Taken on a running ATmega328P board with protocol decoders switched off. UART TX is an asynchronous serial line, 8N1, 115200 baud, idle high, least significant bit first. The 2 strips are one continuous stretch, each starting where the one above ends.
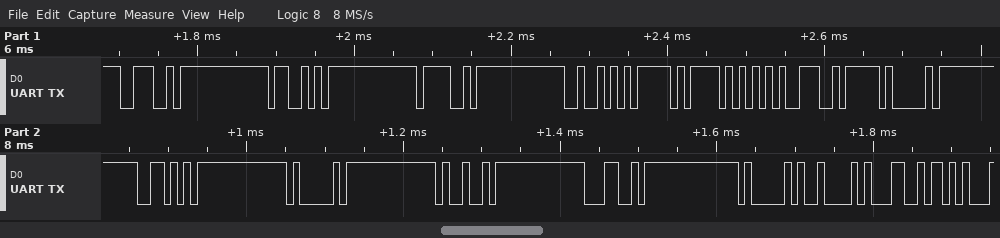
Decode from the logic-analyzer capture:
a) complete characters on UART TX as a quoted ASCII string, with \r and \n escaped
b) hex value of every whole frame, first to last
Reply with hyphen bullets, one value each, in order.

- "NSOR_UNAVAILABL"
- 0x4E 0x53 0x4F 0x52 0x5F 0x55 0x4E 0x41 0x56 0x41 0x49 0x4C 0x41 0x42 0x4C
